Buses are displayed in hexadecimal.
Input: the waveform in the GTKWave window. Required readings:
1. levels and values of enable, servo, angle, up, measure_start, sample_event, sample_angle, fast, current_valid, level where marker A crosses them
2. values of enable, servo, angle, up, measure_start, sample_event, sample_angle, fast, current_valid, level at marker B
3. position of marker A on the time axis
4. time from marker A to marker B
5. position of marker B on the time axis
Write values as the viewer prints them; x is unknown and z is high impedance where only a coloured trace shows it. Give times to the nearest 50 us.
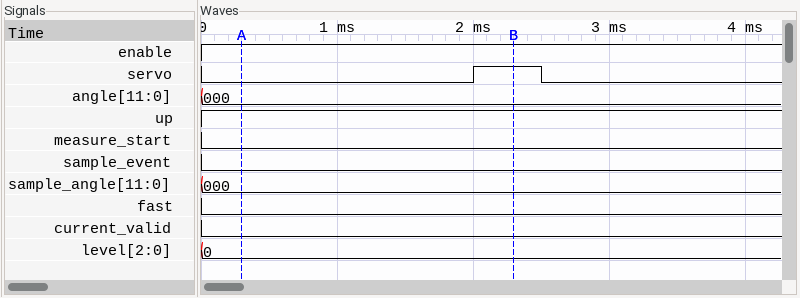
enable=1, servo=0, angle=000, up=1, measure_start=0, sample_event=0, sample_angle=000, fast=0, current_valid=0, level=0
enable=1, servo=1, angle=000, up=1, measure_start=0, sample_event=0, sample_angle=000, fast=0, current_valid=0, level=0
300 us
2000 us
2300 us
